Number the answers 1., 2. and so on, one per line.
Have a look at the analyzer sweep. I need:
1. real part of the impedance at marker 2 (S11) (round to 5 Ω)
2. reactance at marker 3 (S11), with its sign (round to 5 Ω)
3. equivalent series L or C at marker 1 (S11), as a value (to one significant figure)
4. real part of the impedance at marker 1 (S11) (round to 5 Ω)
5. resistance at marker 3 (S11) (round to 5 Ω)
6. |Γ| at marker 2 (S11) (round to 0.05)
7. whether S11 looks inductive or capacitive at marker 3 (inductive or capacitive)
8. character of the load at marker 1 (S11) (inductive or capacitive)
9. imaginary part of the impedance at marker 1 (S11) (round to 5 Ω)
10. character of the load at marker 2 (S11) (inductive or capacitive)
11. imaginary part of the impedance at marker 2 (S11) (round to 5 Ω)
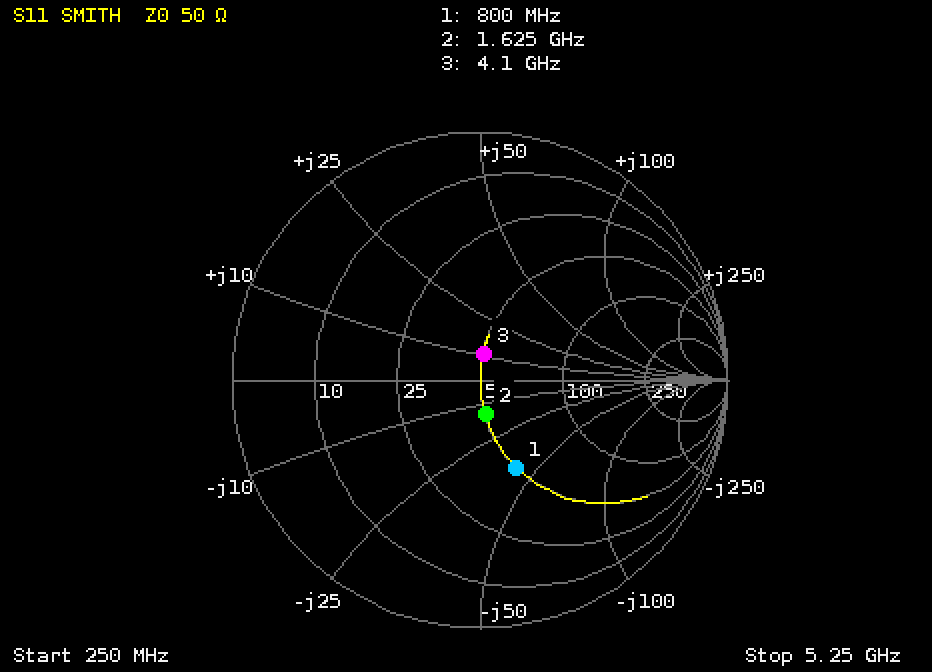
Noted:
1. 50 Ω
2. +10 Ω
3. 5 pF
4. 50 Ω
5. 50 Ω
6. 0.15
7. inductive
8. capacitive
9. -40 Ω
10. capacitive
11. -15 Ω
